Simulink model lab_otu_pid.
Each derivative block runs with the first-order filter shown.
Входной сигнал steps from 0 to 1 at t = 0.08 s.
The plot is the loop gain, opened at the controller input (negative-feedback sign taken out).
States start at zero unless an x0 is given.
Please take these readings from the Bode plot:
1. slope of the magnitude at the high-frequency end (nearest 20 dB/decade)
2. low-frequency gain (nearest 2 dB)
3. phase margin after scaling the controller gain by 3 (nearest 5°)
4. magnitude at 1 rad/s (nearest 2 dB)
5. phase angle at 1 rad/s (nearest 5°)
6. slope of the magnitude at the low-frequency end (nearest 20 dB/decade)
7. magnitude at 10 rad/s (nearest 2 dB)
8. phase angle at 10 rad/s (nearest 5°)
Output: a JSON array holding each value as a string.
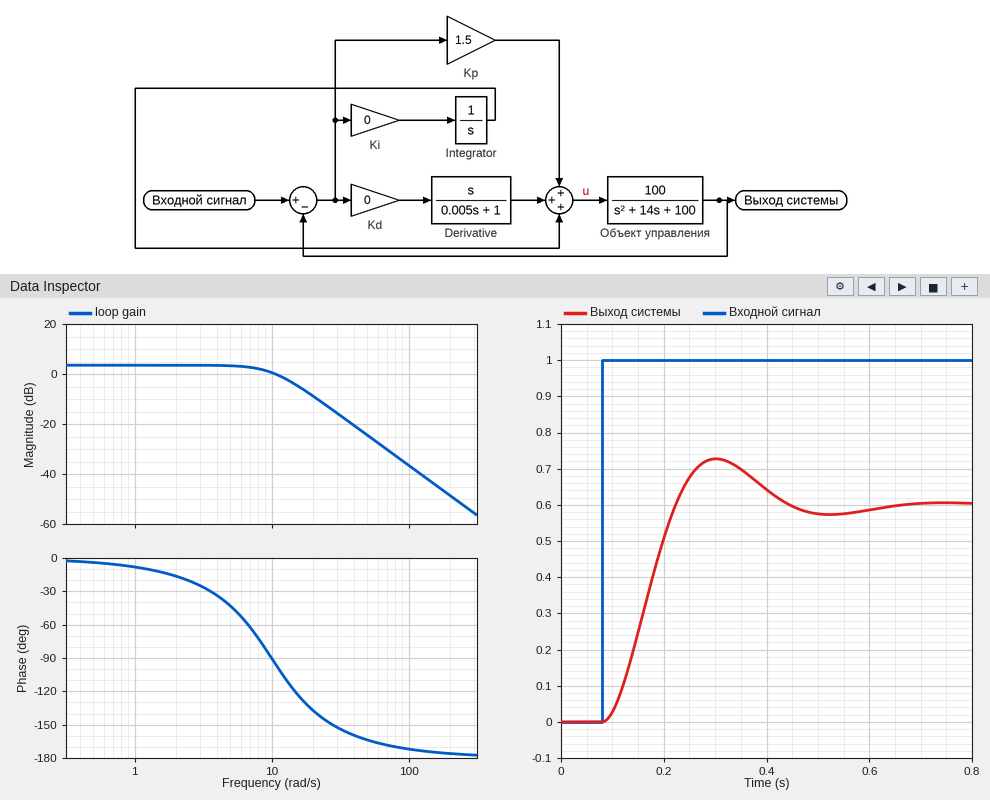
["-40 dB/decade", "4 dB", "40°", "4 dB", "-10°", "0 dB/decade", "0 dB", "-90°"]
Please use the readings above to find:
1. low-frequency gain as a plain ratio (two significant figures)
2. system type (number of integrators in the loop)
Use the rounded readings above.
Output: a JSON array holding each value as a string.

["1.6", "0"]
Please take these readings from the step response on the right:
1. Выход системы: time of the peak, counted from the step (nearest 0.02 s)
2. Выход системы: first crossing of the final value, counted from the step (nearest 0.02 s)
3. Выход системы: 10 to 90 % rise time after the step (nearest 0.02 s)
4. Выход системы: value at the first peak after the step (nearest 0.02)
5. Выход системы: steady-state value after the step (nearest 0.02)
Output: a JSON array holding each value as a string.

["0.22 s", "0.14 s", "0.10 s", "0.72", "0.60"]
